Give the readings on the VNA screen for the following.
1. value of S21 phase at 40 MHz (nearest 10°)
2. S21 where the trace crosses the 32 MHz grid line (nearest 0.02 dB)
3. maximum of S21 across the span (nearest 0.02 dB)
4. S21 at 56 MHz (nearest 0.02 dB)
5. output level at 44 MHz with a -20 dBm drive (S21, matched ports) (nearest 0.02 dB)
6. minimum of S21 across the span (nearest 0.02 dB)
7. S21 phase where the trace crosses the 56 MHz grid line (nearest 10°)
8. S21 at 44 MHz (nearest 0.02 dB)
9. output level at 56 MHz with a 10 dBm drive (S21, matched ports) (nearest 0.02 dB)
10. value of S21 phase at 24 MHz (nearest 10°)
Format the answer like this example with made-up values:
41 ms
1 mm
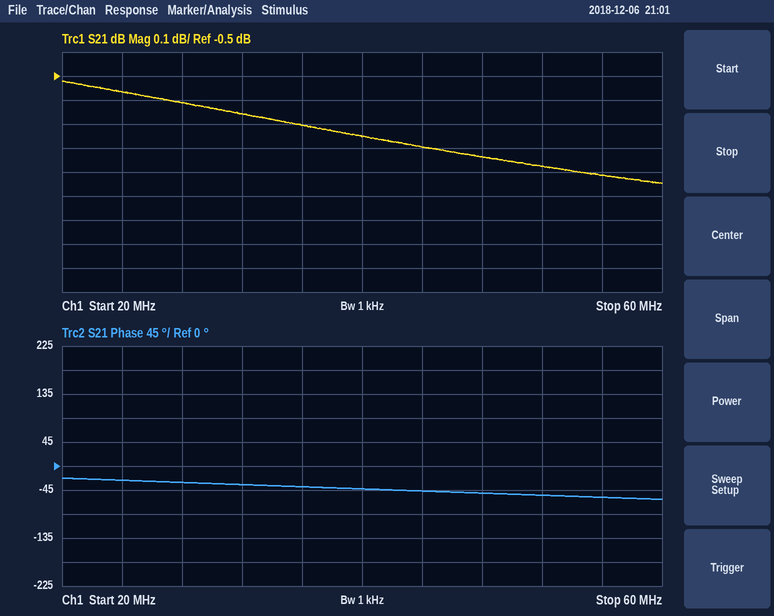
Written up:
-40°
-0.66 dB
-0.52 dB
-0.92 dB
-20.80 dBm
-0.94 dB
-60°
-0.80 dB
9.08 dBm
-30°
